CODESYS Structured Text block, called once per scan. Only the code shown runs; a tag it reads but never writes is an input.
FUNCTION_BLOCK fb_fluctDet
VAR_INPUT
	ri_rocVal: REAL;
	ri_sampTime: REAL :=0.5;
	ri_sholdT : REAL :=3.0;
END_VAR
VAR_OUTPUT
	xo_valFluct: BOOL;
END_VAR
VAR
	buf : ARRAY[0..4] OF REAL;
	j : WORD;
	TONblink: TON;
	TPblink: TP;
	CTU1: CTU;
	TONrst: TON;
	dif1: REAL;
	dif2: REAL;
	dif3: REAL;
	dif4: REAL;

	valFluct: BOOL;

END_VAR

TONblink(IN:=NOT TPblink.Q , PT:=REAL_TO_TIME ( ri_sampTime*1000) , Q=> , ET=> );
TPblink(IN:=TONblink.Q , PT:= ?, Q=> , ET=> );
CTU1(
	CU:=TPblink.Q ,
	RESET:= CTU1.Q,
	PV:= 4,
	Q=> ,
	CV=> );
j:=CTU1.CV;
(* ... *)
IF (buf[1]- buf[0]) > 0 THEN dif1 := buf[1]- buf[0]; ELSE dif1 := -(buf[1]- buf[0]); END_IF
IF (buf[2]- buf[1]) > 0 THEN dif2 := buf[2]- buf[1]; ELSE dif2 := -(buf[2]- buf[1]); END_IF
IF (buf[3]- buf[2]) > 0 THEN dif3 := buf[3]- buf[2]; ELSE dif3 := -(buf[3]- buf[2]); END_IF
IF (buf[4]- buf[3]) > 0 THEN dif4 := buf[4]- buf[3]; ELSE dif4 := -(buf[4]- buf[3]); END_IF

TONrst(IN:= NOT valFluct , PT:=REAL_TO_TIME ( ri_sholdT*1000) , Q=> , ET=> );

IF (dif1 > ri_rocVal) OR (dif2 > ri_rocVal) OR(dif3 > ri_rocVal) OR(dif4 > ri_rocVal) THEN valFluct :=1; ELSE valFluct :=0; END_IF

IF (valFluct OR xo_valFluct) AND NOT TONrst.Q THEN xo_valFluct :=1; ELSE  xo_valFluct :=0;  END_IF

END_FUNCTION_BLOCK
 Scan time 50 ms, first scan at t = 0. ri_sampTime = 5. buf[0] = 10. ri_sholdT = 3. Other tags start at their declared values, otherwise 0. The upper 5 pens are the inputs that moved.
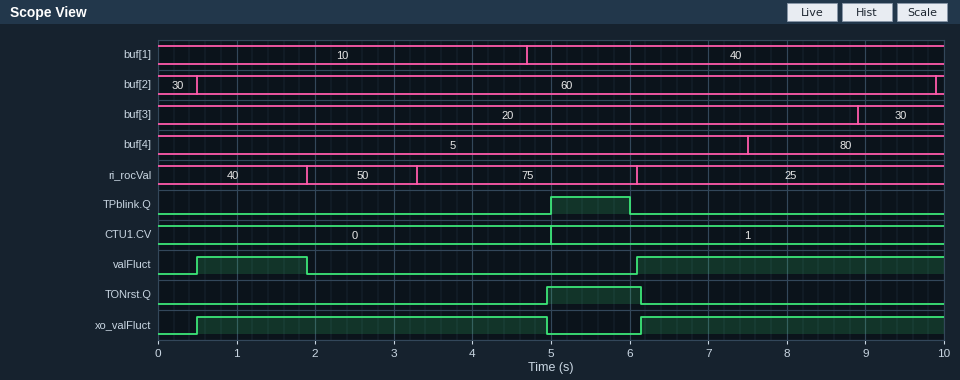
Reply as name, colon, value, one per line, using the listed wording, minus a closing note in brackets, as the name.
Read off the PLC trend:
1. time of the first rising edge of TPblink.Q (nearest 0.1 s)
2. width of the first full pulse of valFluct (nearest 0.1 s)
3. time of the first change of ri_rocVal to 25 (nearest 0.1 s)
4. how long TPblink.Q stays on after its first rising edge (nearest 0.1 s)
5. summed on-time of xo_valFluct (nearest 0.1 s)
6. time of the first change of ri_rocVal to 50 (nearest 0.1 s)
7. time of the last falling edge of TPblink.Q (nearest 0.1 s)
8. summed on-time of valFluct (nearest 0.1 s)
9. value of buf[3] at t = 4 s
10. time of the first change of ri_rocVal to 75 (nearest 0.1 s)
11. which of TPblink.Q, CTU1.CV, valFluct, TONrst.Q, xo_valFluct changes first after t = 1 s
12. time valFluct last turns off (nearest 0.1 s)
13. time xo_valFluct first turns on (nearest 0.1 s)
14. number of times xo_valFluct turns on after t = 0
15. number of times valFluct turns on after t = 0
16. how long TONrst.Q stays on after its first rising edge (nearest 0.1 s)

time of the first rising edge of TPblink.Q: 5.0 s
width of the first full pulse of valFluct: 1.4 s
time of the first change of ri_rocVal to 25: 6.1 s
how long TPblink.Q stays on after its first rising edge: 1.0 s
summed on-time of xo_valFluct: 8.3 s
time of the first change of ri_rocVal to 50: 1.9 s
time of the last falling edge of TPblink.Q: 6.0 s
summed on-time of valFluct: 5.3 s
value of buf[3] at t = 4 s: 20
time of the first change of ri_rocVal to 75: 3.3 s
which of TPblink.Q, CTU1.CV, valFluct, TONrst.Q, xo_valFluct changes first after t = 1 s: valFluct
time valFluct last turns off: 1.9 s
time xo_valFluct first turns on: 0.5 s
number of times xo_valFluct turns on after t = 0: 2
number of times valFluct turns on after t = 0: 2
how long TONrst.Q stays on after its first rising edge: 1.2 s
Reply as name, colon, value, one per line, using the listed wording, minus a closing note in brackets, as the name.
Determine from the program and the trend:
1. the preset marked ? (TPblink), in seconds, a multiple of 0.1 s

the preset marked ? (TPblink), in seconds, a multiple of 0.1 s: 1.0 s
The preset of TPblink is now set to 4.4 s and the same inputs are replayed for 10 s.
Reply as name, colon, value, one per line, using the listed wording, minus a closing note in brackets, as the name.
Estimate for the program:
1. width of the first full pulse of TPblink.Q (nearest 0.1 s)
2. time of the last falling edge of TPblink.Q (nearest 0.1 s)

width of the first full pulse of TPblink.Q: 4.4 s
time of the last falling edge of TPblink.Q: 9.4 s
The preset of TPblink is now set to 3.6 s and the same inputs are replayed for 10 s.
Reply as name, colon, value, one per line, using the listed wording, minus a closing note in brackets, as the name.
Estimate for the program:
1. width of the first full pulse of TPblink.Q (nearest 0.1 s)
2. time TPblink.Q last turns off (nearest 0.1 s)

width of the first full pulse of TPblink.Q: 3.6 s
time TPblink.Q last turns off: 8.6 s
